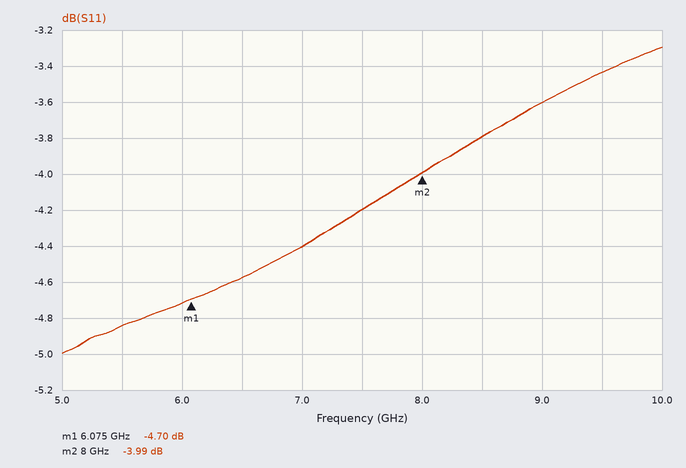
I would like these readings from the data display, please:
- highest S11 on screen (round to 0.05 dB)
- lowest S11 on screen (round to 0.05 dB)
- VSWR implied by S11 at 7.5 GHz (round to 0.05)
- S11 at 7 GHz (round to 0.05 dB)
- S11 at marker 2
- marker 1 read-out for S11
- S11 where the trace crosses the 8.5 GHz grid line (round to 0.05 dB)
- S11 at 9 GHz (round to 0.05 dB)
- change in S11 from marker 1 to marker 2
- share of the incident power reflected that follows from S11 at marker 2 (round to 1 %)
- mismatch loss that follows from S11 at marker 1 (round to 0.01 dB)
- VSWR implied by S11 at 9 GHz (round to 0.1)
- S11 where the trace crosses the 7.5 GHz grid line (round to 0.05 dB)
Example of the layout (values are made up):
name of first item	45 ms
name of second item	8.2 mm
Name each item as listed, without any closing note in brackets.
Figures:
highest S11 on screen	-3.30 dB
lowest S11 on screen	-5.00 dB
VSWR implied by S11 at 7.5 GHz	4.20
S11 at 7 GHz	-4.40 dB
S11 at marker 2	-3.99 dB
marker 1 read-out for S11	-4.70 dB
S11 where the trace crosses the 8.5 GHz grid line	-3.80 dB
S11 at 9 GHz	-3.60 dB
change in S11 from marker 1 to marker 2	0.71 dB
share of the incident power reflected that follows from S11 at marker 2	40 %
mismatch loss that follows from S11 at marker 1	1.80 dB
VSWR implied by S11 at 9 GHz	4.9
S11 where the trace crosses the 7.5 GHz grid line	-4.20 dB
